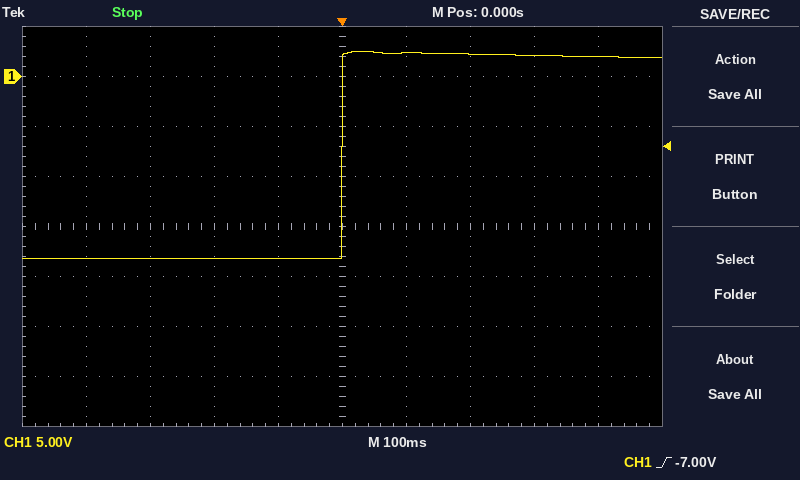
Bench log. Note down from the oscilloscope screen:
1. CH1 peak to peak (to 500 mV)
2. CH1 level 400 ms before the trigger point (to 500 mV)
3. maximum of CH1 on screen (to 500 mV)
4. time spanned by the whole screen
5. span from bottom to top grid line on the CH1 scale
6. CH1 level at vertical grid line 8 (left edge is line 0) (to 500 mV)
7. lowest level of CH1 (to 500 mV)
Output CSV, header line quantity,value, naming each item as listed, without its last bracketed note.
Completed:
quantity,value
CH1 peak to peak,20.5 V
CH1 level 400 ms before the trigger point,-18.0 V
maximum of CH1 on screen,2.5 V
time spanned by the whole screen,1 s
span from bottom to top grid line on the CH1 scale,40 V
CH1 level at vertical grid line 8 (left edge is line 0),2.0 V
lowest level of CH1,-18.0 V
